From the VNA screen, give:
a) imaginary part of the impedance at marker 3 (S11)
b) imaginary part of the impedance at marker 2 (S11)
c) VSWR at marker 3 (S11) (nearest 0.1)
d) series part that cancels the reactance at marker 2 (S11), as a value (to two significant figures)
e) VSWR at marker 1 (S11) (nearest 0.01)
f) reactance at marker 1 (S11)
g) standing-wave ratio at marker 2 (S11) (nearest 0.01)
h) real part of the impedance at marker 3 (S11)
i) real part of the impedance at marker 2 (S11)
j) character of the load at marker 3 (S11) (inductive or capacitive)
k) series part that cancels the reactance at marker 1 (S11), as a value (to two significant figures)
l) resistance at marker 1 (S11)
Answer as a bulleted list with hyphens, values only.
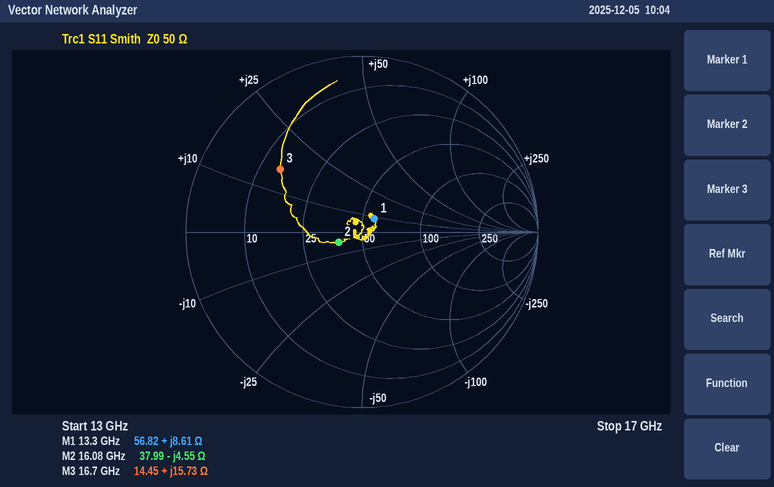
- +15.73 Ω
- -4.55 Ω
- 3.8
- 45 pH
- 1.23
- +8.61 Ω
- 1.34
- 14.45 Ω
- 37.99 Ω
- inductive
- 1.4 pF
- 56.82 Ω
